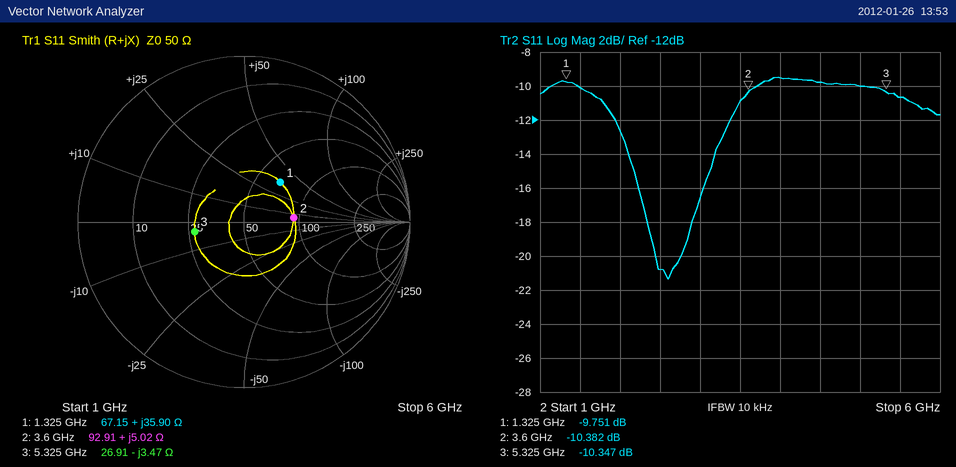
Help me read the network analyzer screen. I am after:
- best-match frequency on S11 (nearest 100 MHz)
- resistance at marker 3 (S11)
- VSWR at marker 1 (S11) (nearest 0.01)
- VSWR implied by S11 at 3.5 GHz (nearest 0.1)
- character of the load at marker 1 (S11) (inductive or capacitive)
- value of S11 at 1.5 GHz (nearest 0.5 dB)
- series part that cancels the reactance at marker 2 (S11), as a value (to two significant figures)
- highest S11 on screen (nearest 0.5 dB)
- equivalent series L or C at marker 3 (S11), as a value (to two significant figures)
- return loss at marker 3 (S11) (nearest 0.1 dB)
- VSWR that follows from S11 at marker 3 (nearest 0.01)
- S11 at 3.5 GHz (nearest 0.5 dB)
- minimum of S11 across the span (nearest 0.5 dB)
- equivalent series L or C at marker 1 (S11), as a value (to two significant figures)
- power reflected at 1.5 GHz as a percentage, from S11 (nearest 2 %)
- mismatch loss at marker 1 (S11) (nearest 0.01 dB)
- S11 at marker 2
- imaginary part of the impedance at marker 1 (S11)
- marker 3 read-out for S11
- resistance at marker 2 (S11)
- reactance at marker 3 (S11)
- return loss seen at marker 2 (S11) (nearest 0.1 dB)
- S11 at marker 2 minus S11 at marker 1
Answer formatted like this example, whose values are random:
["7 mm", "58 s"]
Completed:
["2.6 GHz", "26.91 Ω", "1.96", "1.8", "inductive", "-10.0 dB", "8.8 pF", "-9.5 dB", "8.6 pF", "10.4 dB", "1.87", "-11.0 dB", "-21.5 dB", "4.3 nH", "10 %", "0.49 dB", "-10.382 dB", "+35.90 Ω", "-10.347 dB", "92.91 Ω", "-3.47 Ω", "10.4 dB", "-0.631 dB"]
